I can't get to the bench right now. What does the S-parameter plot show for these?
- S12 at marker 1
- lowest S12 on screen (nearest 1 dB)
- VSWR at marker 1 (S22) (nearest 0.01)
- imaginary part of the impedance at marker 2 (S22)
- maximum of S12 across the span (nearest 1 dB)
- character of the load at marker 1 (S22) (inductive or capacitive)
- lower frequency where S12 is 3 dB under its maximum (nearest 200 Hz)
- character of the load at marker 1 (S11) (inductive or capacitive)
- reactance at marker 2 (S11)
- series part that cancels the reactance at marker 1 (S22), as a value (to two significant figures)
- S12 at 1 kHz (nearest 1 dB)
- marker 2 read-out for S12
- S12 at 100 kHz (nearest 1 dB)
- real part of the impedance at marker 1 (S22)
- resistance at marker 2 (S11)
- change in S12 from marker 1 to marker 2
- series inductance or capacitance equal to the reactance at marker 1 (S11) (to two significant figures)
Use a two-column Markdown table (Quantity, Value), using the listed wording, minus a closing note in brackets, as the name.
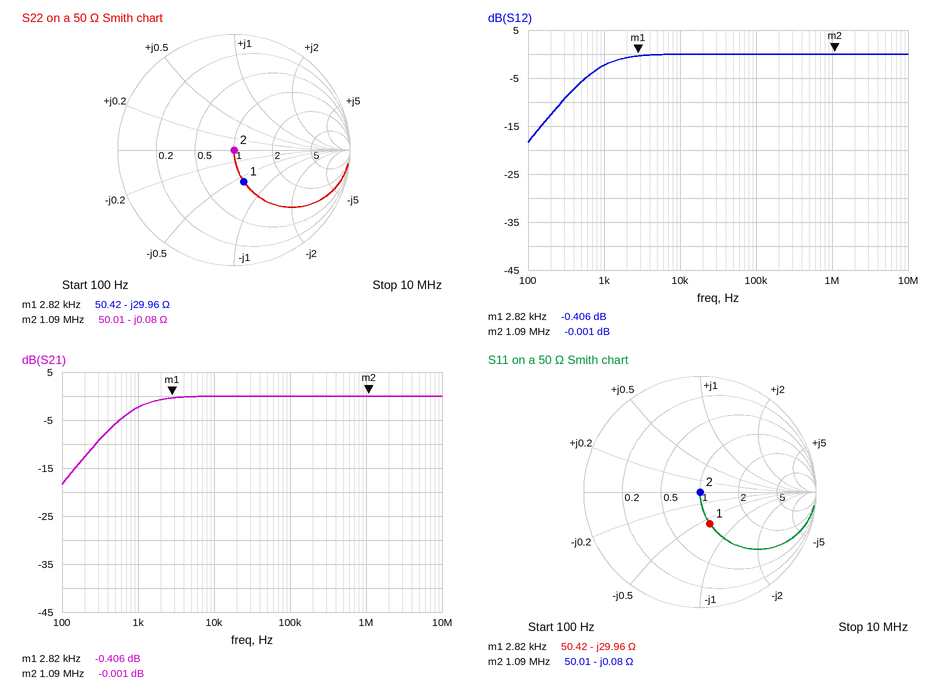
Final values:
| Quantity | Value |
|---|---|
| S12 at marker 1 | -0.406 dB |
| lowest S12 on screen | -18 dB |
| VSWR at marker 1 (S22) | 1.80 |
| imaginary part of the impedance at marker 2 | -0.08 Ω |
| maximum of S12 across the span | 0 dB |
| character of the load at marker 1 (S22) | capacitive |
| lower frequency where S12 is 3 dB under its maximum | 800 Hz |
| character of the load at marker 1 (S11) | capacitive |
| reactance at marker 2 | -0.08 Ω |
| series part that cancels the reactance at marker 1 (S22), as a value | 1.7 mH |
| S12 at 1 kHz | -2 dB |
| marker 2 read-out for S12 | -0.001 dB |
| S12 at 100 kHz | 0 dB |
| real part of the impedance at marker 1 | 50.42 Ω |
| resistance at marker 2 | 50.01 Ω |
| change in S12 from marker 1 to marker 2 | 0.405 dB |
| series inductance or capacitance equal to the reactance at marker 1 (S11) | 1.9 µF |
